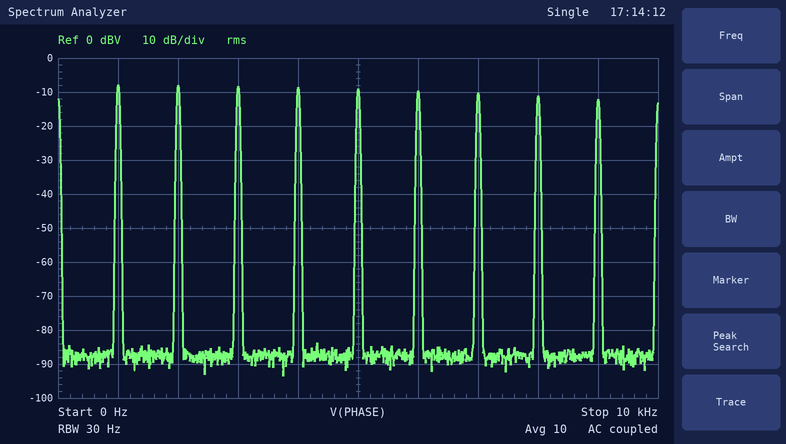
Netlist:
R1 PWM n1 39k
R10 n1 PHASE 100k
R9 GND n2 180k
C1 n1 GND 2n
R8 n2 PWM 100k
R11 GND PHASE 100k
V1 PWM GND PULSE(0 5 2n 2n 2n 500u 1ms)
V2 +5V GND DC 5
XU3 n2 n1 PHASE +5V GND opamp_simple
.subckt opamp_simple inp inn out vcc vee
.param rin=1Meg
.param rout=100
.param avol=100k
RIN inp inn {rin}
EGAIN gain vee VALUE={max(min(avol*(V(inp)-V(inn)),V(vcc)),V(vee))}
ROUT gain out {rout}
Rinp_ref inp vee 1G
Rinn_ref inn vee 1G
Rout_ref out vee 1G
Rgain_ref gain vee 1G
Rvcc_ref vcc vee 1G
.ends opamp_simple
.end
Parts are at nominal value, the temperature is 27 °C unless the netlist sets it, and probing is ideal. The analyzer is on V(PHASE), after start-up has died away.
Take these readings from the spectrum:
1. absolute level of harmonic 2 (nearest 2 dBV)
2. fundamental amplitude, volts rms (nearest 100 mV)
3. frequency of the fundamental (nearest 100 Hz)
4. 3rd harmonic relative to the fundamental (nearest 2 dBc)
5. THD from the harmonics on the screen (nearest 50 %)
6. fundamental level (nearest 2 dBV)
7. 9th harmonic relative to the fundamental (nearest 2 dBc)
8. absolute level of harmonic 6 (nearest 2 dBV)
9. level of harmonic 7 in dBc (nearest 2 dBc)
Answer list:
-8 dBV
400 mV
1.0 kHz
0 dBc
250 %
-8 dBV
-4 dBc
-10 dBV
-2 dBc
